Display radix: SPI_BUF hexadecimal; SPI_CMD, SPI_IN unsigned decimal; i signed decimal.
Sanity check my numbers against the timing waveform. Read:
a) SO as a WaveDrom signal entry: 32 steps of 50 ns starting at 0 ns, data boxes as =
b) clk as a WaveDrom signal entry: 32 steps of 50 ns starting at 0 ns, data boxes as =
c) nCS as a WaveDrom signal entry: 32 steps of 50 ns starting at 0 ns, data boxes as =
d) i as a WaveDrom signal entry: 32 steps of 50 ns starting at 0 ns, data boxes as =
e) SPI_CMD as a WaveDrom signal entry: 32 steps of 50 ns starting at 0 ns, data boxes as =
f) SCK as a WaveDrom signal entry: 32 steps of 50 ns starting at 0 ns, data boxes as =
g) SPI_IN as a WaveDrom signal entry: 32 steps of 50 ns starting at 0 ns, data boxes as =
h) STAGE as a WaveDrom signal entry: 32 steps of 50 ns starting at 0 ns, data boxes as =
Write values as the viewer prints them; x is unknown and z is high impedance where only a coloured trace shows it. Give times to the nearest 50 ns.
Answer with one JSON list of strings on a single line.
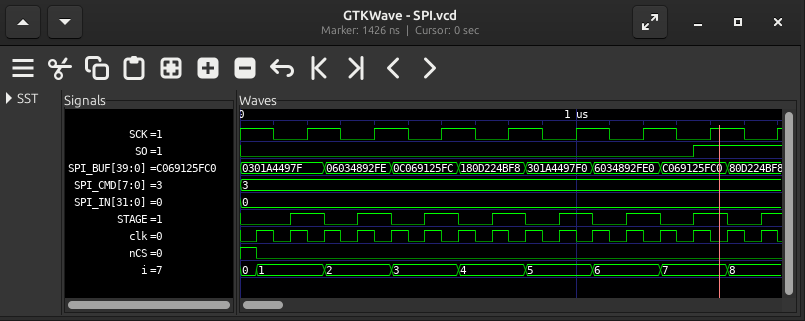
["{name: 'SO', wave: '0..........................1....'}", "{name: 'clk', wave: '01010101010101010101010101010101'}", "{name: 'nCS', wave: '10..............................'}", "{name: 'i', wave: '==...=...=...=...=...=...=...=..', data: '0 1 2 3 4 5 6 7 8'}", "{name: 'SPI_CMD', wave: '=...............................', data: '3'}", "{name: 'SCK', wave: '1.0.1.0.1.0.1.0.1.0.1.0.1.0.1.0.'}", "{name: 'SPI_IN', wave: '=...............................', data: '0'}", "{name: 'STAGE', wave: '0..1.0.1.0.1.0.1.0.1.0.1.0.1.0.1'}"]
